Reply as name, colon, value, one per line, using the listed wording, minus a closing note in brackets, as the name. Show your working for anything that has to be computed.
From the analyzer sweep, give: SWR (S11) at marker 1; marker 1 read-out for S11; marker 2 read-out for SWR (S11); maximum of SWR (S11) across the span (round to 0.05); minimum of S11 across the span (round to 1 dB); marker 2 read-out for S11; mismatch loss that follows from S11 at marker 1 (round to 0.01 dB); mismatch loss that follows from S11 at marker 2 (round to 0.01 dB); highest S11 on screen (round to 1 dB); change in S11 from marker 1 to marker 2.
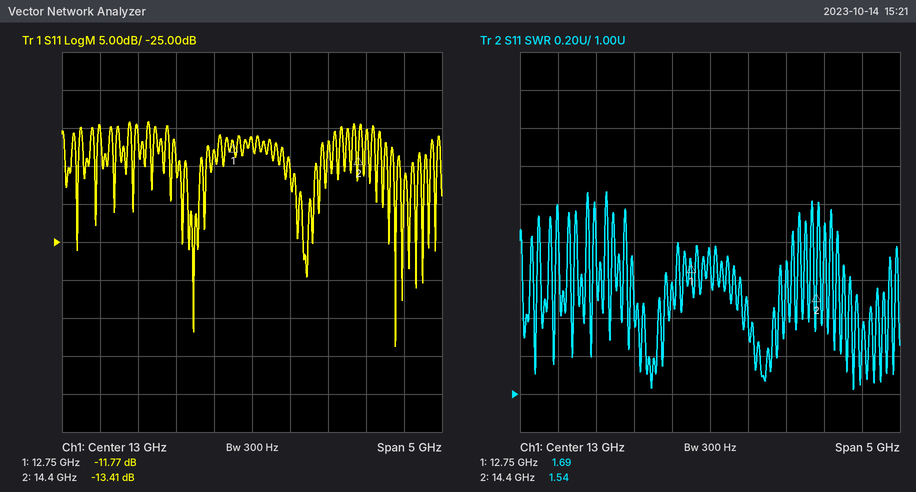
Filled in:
SWR (S11) at marker 1: 1.69
marker 1 read-out for S11: -11.77 dB
marker 2 read-out for SWR: 1.54
maximum of SWR (S11) across the span: 2.05
minimum of S11 across the span: -39 dB
marker 2 read-out for S11: -13.41 dB
mismatch loss that follows from S11 at marker 1: −10 log10(1 − 10^(-11.77/10)) ≈ 0.30 dB
mismatch loss that follows from S11 at marker 2: −10 log10(1 − 10^(-13.41/10)) ≈ 0.20 dB
highest S11 on screen: -9 dB
change in S11 from marker 1 to marker 2: -13.41 − (-11.77) = -1.64 dB
